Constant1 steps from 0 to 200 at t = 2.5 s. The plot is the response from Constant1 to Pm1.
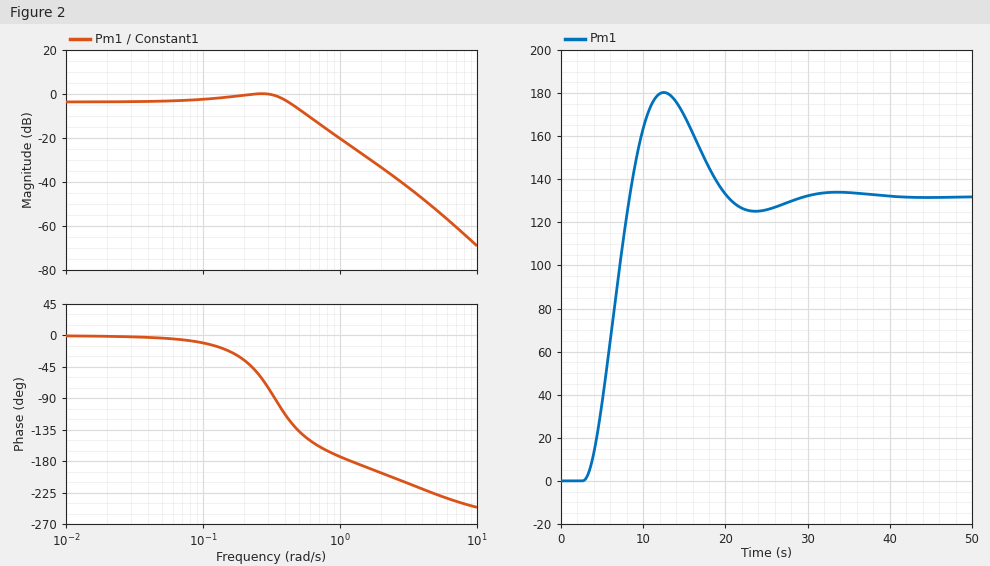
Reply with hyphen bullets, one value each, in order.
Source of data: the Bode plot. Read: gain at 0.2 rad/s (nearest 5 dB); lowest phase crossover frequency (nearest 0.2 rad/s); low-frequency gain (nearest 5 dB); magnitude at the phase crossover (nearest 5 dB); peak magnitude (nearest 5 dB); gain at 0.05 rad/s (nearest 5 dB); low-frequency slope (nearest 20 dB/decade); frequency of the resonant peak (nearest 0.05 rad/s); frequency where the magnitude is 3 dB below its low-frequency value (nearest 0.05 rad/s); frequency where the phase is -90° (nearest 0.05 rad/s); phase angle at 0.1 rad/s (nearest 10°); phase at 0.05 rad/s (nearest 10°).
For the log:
- 0 dB
- 1.2 rad/s
- -5 dB
- -25 dB
- 0 dB
- -5 dB
- 0 dB/decade
- 0.25 rad/s
- 0.50 rad/s
- 0.35 rad/s
- -10°
- 0°
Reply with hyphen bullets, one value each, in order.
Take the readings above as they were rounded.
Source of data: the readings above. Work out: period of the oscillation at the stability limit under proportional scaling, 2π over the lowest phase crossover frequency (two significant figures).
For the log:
- 5.2 s
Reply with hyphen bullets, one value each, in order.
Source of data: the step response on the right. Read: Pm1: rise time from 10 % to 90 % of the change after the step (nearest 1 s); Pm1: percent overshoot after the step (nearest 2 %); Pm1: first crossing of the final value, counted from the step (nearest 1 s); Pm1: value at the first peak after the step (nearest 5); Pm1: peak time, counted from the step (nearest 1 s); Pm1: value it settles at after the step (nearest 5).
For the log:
- 4 s
- 36 %
- 6 s
- 180
- 10 s
- 130
